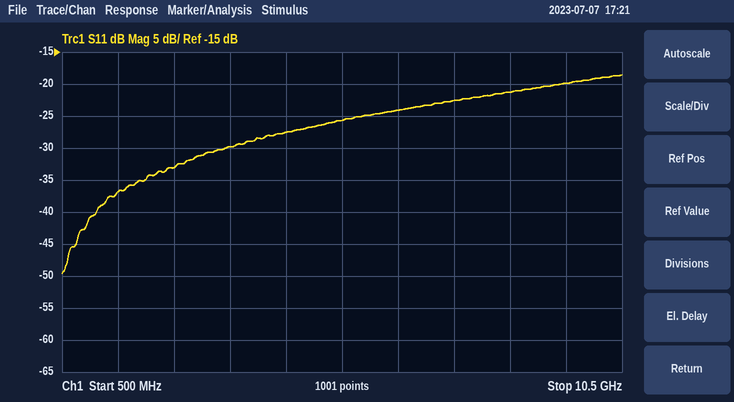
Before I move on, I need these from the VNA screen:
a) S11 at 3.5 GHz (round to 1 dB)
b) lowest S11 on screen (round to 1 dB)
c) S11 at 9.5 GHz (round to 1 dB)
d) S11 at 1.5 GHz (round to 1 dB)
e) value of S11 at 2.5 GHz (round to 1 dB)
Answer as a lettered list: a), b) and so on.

a) -30 dB
b) -50 dB
c) -20 dB
d) -37 dB
e) -33 dB
